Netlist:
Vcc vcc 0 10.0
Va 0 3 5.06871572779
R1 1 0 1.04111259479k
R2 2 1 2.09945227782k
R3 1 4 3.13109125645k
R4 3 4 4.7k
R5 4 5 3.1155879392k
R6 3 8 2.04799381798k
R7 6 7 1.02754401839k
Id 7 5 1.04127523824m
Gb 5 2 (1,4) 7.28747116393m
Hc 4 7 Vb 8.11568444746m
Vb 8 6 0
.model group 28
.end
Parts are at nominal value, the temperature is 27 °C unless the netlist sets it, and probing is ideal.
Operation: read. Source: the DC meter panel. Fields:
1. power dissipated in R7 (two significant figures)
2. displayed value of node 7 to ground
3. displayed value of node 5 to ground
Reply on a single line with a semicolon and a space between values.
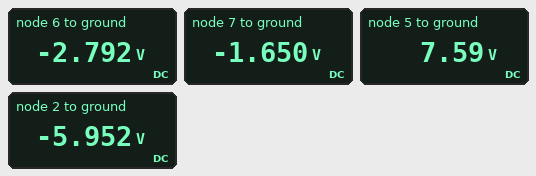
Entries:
1.3 mW; -1.650 V; 7.59 V
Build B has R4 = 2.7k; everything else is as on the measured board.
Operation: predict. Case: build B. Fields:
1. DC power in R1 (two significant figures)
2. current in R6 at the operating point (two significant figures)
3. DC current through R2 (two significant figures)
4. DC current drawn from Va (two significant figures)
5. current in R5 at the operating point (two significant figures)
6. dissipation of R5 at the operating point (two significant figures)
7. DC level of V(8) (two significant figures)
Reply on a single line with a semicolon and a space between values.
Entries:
4.9 mW; 1.0 mA; 2.3 mA; 2.2 mA; 3.3 mA; 34 mW; -3.0 V
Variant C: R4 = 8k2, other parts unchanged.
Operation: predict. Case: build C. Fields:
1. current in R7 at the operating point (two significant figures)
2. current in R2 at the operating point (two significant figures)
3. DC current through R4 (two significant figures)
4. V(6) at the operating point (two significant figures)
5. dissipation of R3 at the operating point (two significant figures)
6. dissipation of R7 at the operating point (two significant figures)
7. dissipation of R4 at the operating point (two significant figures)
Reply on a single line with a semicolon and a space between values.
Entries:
1.2 mA; 1.7 mA; 440 µA; -2.7 V; 17 µW; 1.4 mW; 1.6 mW
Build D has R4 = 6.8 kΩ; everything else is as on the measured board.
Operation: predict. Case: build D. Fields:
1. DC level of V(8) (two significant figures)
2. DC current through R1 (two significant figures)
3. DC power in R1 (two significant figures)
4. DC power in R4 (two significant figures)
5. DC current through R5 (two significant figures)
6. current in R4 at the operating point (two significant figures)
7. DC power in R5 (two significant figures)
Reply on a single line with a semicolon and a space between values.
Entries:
-2.7 V; 1.7 mA; 2.9 mW; 1.9 mW; 2.8 mA; 520 µA; 24 mW
